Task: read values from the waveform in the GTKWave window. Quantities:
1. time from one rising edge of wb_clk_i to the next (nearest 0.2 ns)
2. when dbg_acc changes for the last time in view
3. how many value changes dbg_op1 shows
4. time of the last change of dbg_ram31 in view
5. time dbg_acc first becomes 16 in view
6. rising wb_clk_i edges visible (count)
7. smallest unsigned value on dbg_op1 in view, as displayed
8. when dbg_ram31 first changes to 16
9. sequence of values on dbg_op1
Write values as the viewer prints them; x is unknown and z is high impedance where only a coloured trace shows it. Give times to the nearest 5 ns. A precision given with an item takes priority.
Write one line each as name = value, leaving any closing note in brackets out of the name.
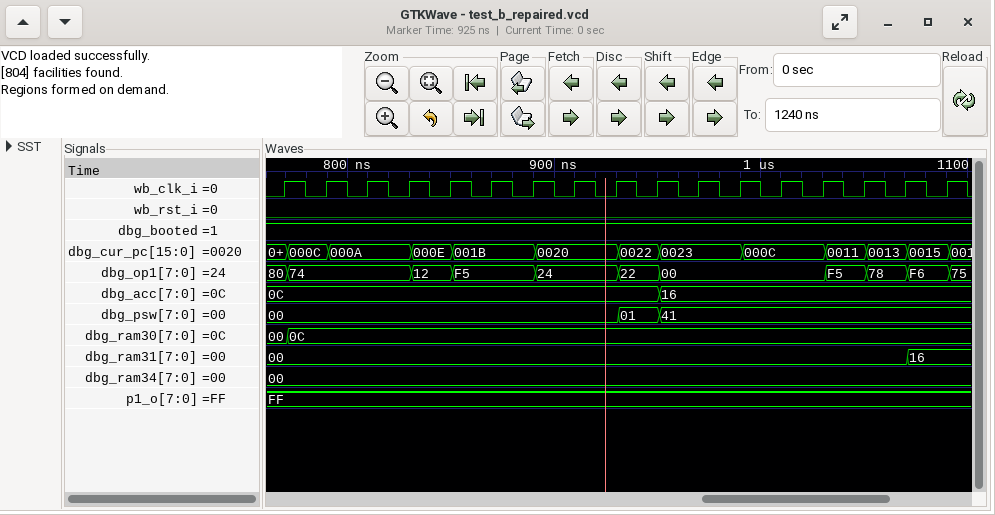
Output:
time from one rising edge of wb_clk_i to the next = 20 ns
when dbg_acc changes for the last time in view = 950 ns
how many value changes dbg_op1 shows = 10
time of the last change of dbg_ram31 in view = 1070 ns
time dbg_acc first becomes 16 in view = 950 ns
rising wb_clk_i edges visible = 17
smallest unsigned value on dbg_op1 in view, as displayed = 00
when dbg_ram31 first changes to 16 = 1070 ns
sequence of values on dbg_op1 = 80, 74, 12, F5, 24, 22, 00, F5, 78, F6, 75
